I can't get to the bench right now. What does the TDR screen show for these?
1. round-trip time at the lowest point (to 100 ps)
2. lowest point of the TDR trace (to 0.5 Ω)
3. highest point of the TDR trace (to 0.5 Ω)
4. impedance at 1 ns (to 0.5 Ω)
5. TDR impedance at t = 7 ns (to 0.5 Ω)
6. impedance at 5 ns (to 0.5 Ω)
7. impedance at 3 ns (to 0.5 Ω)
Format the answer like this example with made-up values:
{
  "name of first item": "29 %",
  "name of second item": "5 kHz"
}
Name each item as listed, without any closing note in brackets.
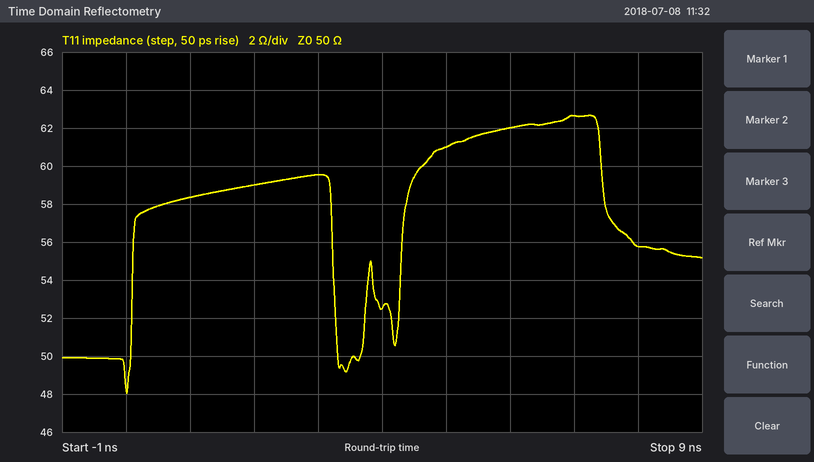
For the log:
{
  "round-trip time at the lowest point": "0.0 ns",
  "lowest point of the TDR trace": "48.0 Ω",
  "highest point of the TDR trace": "62.5 Ω",
  "impedance at 1 ns": "58.5 Ω",
  "TDR impedance at t = 7 ns": "62.5 Ω",
  "impedance at 5 ns": "61.0 Ω",
  "impedance at 3 ns": "59.5 Ω"
}
